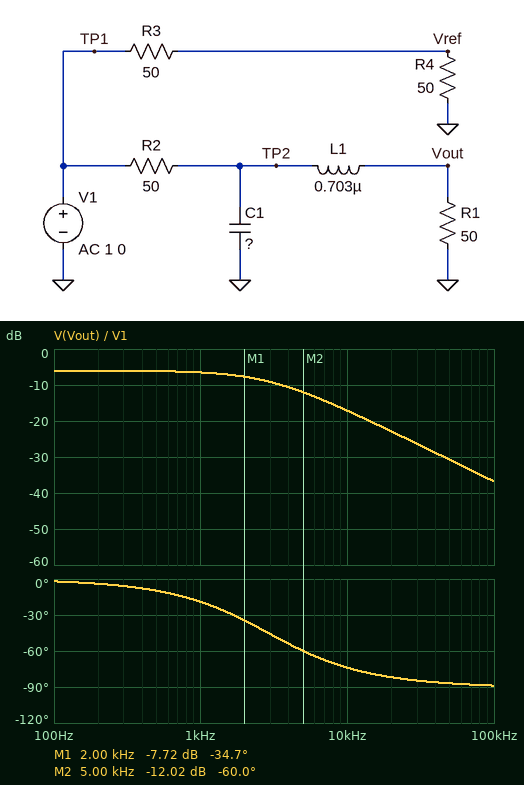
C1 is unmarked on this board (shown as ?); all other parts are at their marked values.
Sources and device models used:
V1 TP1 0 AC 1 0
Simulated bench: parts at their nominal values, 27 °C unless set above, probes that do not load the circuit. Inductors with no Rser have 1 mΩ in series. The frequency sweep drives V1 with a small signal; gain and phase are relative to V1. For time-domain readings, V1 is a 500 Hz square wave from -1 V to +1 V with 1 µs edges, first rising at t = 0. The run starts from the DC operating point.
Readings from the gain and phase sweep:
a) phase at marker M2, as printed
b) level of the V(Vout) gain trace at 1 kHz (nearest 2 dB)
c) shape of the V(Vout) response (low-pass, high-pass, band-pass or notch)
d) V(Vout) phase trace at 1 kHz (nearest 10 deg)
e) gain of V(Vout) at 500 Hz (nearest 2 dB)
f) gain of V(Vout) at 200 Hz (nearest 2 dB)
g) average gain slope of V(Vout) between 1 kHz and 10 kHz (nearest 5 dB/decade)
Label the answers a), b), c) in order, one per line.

a) -60.0 deg
b) -6 dB
c) low-pass
d) -20 deg
e) -6 dB
f) -6 dB
g) -10 dB/decade
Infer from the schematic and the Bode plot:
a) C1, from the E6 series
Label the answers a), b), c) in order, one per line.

a) 2.2 µF
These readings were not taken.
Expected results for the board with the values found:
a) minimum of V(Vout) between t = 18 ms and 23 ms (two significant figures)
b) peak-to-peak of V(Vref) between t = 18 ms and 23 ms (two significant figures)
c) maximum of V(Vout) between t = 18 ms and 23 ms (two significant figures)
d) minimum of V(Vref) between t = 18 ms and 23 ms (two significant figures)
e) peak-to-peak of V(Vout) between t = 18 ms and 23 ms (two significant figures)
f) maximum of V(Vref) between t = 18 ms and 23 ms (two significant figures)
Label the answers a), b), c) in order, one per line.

a) -500 mV
b) 1.0 V
c) 500 mV
d) -500 mV
e) 1.0 V
f) 500 mV
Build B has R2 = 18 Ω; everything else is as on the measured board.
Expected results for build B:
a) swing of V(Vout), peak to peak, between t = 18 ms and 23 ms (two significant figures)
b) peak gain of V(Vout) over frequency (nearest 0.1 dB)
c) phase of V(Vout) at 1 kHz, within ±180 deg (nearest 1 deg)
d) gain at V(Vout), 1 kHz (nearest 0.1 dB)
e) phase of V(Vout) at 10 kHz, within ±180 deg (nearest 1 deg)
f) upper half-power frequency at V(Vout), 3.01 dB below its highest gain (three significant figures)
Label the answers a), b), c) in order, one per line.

a) 1.5 V
b) -2.7 dB
c) -10 deg
d) -2.8 dB
e) -61 deg
f) 5.47 kHz
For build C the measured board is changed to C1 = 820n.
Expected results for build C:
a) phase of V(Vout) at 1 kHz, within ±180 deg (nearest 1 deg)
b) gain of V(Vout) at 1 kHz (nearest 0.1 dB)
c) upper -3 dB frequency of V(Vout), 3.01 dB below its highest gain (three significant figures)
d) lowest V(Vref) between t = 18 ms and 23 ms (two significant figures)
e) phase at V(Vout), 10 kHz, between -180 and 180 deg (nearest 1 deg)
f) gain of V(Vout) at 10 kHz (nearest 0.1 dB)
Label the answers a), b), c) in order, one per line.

a) -7 deg
b) -6.1 dB
c) 7.77 kHz
d) -500 mV
e) -52 deg
f) -10.3 dB
